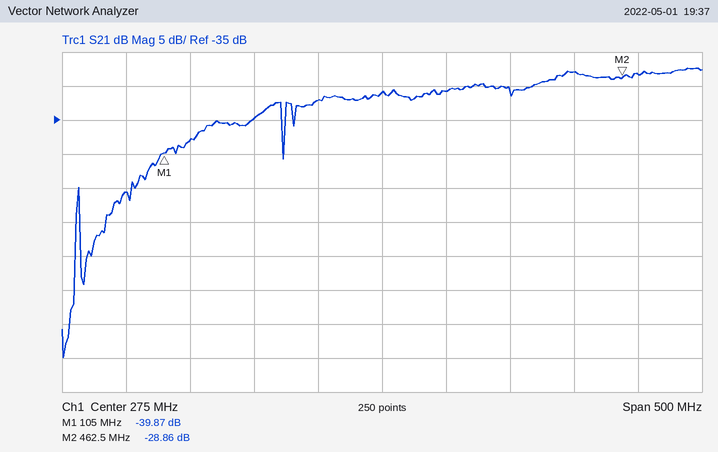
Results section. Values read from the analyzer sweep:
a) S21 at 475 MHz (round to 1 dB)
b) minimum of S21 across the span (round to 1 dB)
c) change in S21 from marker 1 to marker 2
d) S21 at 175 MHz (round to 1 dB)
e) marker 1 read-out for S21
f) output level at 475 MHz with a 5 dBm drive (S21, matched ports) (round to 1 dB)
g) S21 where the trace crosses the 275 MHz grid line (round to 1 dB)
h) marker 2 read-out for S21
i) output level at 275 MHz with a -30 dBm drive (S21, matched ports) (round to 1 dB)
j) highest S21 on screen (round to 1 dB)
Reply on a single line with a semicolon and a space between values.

-28 dB; -70 dB; 11.01 dB; -35 dB; -39.87 dB; -23 dBm; -31 dB; -28.86 dB; -61 dBm; -27 dB
